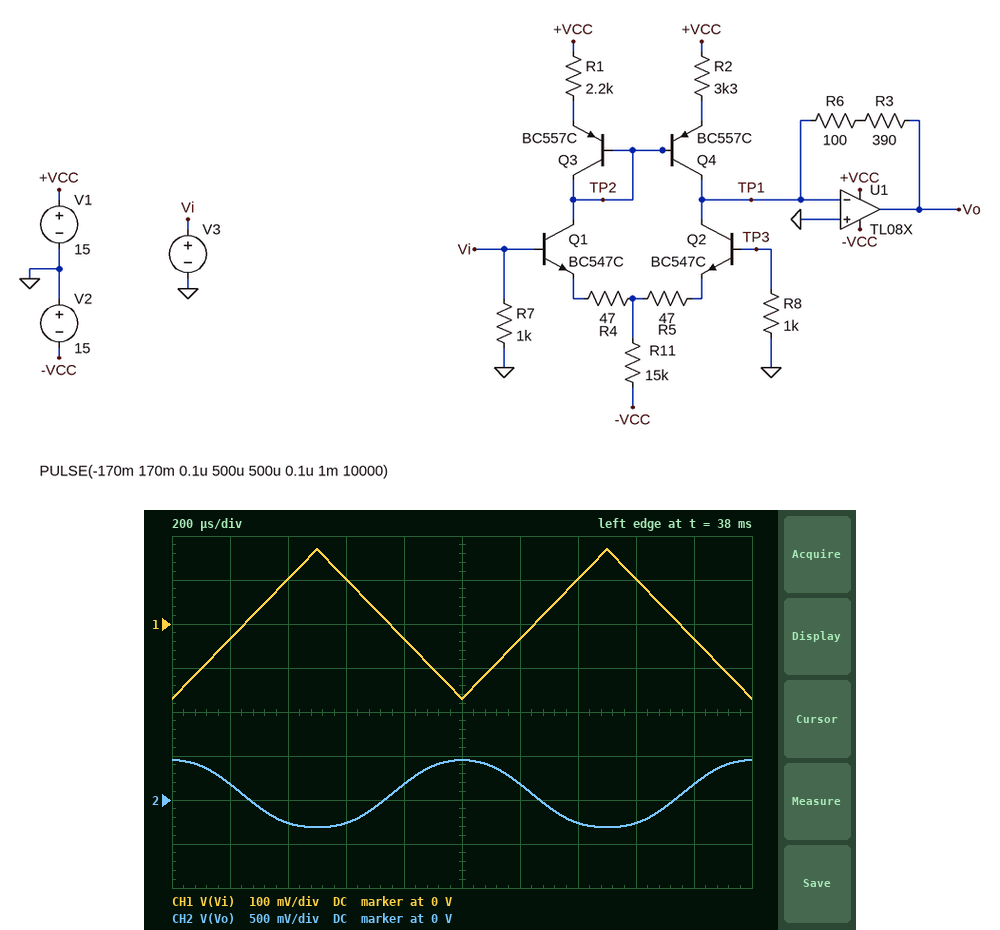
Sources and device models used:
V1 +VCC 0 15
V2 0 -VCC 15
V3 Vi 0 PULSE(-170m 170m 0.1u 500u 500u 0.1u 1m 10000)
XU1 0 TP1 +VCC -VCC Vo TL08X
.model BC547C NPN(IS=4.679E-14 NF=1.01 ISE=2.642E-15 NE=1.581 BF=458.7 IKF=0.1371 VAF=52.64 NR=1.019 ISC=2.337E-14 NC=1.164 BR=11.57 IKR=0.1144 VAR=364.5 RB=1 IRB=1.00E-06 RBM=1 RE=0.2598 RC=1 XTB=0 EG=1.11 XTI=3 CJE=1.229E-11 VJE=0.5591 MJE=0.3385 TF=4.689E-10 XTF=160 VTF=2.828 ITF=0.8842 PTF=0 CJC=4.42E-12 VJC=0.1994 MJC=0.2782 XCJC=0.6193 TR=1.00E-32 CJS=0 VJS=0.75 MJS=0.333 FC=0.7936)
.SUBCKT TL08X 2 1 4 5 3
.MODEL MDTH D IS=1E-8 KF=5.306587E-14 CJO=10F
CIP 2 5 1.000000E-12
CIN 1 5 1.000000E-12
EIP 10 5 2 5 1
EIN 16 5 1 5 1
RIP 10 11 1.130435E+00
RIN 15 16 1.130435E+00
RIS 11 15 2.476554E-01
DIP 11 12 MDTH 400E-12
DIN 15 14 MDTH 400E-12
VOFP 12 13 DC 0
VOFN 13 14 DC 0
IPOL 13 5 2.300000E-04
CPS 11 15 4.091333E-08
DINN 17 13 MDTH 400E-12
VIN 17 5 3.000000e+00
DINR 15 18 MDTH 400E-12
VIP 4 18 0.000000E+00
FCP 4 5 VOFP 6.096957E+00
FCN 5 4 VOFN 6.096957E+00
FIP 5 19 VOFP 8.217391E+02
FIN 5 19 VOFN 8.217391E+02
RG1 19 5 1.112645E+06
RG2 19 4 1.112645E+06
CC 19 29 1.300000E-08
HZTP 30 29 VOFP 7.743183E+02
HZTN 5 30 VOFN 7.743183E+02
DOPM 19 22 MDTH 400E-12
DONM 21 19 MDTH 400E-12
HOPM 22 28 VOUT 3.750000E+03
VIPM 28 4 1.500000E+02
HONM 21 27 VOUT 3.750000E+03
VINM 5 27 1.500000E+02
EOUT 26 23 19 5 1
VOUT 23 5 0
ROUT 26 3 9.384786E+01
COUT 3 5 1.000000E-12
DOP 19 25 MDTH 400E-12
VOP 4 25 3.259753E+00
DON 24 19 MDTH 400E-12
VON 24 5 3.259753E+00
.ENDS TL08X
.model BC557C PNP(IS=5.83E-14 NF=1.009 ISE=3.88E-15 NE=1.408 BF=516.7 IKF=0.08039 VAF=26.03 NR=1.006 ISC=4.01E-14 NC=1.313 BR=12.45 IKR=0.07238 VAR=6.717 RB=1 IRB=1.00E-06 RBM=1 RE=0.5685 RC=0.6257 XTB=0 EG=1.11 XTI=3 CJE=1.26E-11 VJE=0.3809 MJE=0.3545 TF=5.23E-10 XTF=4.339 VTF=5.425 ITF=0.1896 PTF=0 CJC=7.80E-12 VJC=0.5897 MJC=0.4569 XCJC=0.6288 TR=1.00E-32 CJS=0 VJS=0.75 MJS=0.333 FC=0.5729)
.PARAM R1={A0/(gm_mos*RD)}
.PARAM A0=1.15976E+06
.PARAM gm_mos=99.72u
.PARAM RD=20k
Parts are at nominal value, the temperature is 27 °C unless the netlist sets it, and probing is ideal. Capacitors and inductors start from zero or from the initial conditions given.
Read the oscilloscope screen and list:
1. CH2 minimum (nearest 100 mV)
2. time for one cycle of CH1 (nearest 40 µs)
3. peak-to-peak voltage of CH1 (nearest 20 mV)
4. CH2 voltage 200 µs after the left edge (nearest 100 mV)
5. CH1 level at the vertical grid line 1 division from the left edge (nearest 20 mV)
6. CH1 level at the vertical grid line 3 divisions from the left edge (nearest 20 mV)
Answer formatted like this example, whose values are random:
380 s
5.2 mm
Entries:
-300 mV
1.00 ms
340 mV
200 mV
-40 mV
100 mV
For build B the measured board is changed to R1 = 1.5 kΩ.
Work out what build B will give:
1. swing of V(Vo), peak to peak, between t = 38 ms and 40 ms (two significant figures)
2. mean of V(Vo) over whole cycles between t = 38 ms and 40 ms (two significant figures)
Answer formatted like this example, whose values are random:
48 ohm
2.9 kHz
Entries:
670 mV
110 mV
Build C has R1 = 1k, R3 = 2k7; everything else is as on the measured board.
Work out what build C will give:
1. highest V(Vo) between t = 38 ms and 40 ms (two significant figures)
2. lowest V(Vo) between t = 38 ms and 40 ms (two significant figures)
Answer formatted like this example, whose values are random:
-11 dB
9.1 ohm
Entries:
2.6 V
-830 mV
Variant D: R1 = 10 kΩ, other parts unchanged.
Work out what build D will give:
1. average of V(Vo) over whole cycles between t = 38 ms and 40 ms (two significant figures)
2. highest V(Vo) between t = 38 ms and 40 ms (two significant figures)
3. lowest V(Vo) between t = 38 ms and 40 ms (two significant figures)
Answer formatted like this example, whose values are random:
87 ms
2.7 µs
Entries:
-500 mV
450 mV
-1.4 V
